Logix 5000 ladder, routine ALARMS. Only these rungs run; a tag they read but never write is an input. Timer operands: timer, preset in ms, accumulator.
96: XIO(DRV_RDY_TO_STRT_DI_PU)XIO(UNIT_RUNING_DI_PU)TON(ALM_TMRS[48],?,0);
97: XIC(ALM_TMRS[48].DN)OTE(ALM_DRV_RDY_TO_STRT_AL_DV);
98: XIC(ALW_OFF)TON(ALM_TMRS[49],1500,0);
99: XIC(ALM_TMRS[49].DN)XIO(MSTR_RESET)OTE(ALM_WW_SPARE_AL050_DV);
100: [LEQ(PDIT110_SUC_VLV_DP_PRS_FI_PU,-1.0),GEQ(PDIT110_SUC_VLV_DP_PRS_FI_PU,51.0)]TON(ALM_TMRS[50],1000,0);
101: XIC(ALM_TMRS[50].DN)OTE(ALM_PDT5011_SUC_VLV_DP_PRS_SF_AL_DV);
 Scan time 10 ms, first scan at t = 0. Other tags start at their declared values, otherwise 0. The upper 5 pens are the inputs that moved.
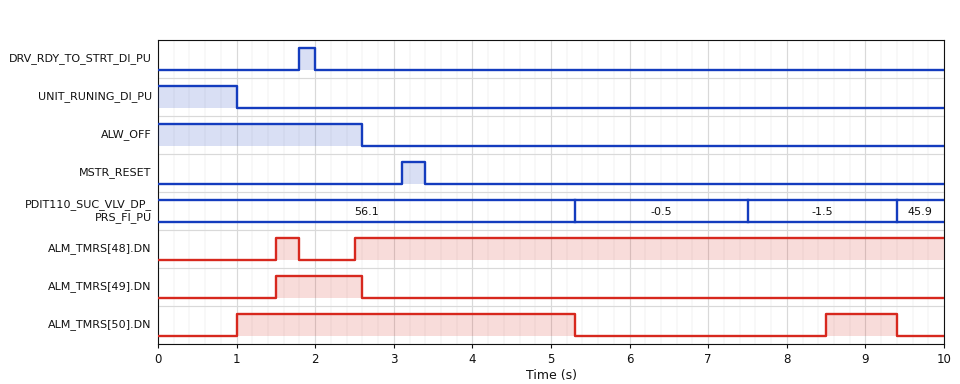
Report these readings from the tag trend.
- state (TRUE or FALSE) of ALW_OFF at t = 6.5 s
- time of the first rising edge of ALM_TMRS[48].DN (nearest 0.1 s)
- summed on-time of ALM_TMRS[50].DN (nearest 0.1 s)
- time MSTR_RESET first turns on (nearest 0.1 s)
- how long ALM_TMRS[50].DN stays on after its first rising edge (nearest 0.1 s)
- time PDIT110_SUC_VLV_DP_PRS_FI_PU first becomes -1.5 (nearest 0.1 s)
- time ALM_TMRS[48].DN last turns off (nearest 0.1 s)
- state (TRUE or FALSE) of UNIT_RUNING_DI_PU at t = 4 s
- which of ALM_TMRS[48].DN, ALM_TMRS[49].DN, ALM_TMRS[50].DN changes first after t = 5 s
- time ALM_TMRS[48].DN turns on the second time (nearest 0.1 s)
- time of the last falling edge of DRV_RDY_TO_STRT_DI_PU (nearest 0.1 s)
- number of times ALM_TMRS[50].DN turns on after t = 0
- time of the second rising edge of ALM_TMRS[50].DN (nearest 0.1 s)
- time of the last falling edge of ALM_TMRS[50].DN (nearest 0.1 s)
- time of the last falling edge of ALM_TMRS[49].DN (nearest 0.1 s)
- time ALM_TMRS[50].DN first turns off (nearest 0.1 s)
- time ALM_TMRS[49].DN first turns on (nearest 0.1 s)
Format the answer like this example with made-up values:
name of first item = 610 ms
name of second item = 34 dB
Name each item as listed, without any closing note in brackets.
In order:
state (TRUE or FALSE) of ALW_OFF at t = 6.5 s = FALSE
time of the first rising edge of ALM_TMRS[48].DN = 1.5 s
summed on-time of ALM_TMRS[50].DN = 5.2 s
time MSTR_RESET first turns on = 3.1 s
how long ALM_TMRS[50].DN stays on after its first rising edge = 4.3 s
time PDIT110_SUC_VLV_DP_PRS_FI_PU first becomes -1.5 = 7.5 s
time ALM_TMRS[48].DN last turns off = 1.8 s
state (TRUE or FALSE) of UNIT_RUNING_DI_PU at t = 4 s = FALSE
which of ALM_TMRS[48].DN, ALM_TMRS[49].DN, ALM_TMRS[50].DN changes first after t = 5 s = ALM_TMRS[50].DN
time ALM_TMRS[48].DN turns on the second time = 2.5 s
time of the last falling edge of DRV_RDY_TO_STRT_DI_PU = 2.0 s
number of times ALM_TMRS[50].DN turns on after t = 0 = 2
time of the second rising edge of ALM_TMRS[50].DN = 8.5 s
time of the last falling edge of ALM_TMRS[50].DN = 9.4 s
time of the last falling edge of ALM_TMRS[49].DN = 2.6 s
time ALM_TMRS[50].DN first turns off = 5.3 s
time ALM_TMRS[49].DN first turns on = 1.5 s
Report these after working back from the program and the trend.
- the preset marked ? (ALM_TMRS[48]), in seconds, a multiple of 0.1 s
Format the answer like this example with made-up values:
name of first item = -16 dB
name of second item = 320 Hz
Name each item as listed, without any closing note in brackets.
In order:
the preset marked ? (ALM_TMRS[48]), in seconds, a multiple of 0.1 s = 0.5 s
